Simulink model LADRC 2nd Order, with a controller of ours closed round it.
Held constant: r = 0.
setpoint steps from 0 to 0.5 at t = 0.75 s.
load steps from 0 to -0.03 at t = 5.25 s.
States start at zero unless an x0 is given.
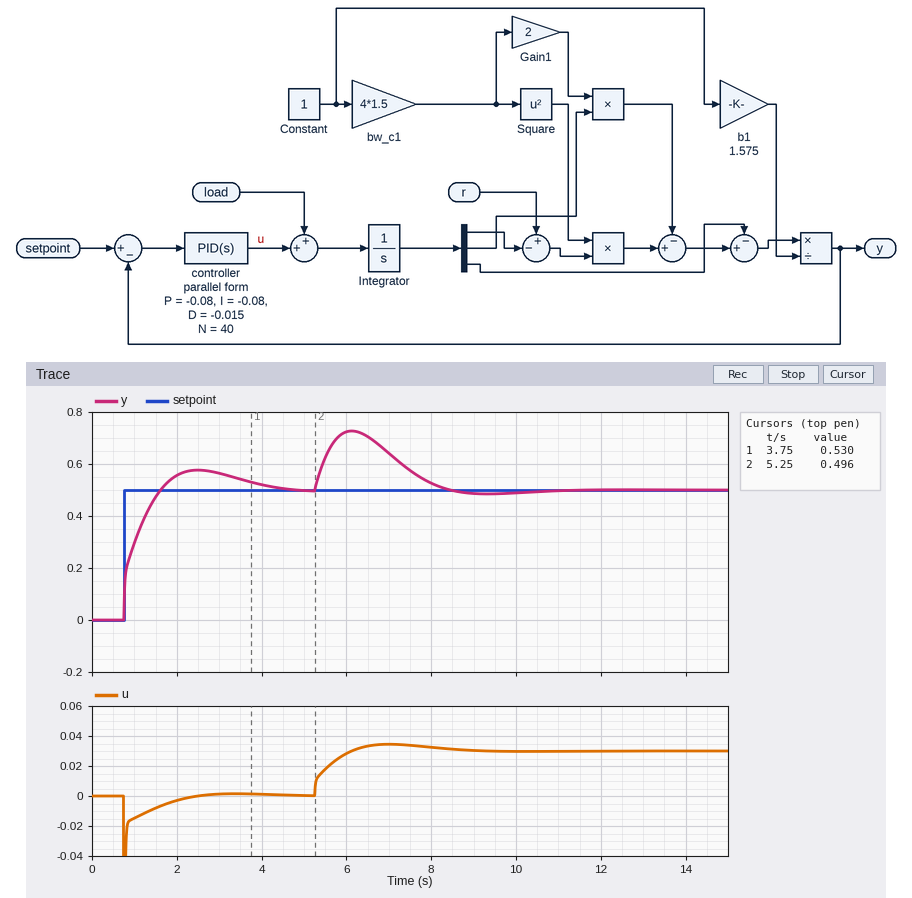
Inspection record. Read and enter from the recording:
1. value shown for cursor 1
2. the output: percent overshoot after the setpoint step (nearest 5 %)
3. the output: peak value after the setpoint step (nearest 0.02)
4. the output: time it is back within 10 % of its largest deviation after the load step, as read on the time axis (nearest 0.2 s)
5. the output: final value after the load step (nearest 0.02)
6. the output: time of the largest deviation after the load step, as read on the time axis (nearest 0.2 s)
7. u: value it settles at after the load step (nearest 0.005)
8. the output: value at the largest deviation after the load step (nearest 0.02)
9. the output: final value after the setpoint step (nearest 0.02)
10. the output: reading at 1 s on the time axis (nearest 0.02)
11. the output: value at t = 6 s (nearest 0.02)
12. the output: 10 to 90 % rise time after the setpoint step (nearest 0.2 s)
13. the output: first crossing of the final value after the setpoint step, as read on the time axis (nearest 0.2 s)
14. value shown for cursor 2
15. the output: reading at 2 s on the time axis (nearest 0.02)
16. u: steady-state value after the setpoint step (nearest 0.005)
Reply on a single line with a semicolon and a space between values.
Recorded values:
0.530; 15 %; 0.58; 8.0 s; 0.50; 6.2 s; 0.030; 0.72; 0.50; 0.30; 0.72; 0.6 s; 1.6 s; 0.496; 0.56; 0.000
